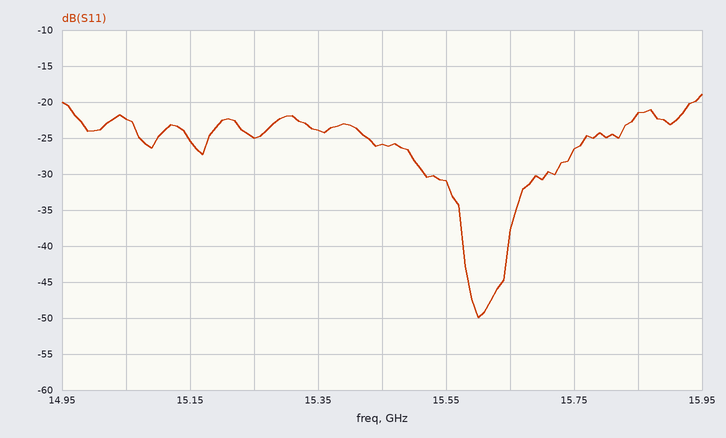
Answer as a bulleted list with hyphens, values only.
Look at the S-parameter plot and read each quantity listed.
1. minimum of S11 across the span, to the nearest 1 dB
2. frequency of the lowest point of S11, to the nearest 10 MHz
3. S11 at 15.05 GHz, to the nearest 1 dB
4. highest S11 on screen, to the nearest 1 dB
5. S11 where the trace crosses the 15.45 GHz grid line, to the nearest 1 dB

- -50 dB
- 15.60 GHz
- -22 dB
- -19 dB
- -26 dB
